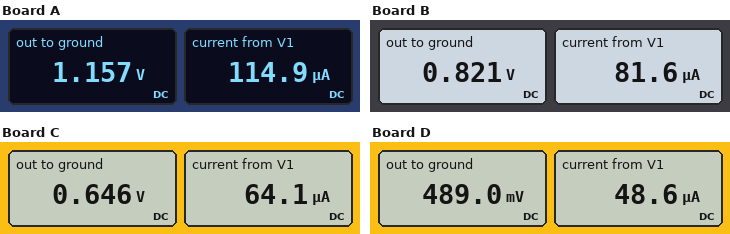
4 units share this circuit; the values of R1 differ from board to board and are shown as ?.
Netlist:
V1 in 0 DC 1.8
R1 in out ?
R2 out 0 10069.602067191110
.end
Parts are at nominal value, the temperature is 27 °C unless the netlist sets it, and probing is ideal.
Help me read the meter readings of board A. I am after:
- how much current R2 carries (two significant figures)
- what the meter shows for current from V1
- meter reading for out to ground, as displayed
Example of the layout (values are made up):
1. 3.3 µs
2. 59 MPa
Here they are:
1. 110 µA
2. 114.9 µA
3. 1.157 V
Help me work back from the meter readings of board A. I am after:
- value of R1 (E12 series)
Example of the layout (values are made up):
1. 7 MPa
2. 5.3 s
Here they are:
1. 5.6 kΩ
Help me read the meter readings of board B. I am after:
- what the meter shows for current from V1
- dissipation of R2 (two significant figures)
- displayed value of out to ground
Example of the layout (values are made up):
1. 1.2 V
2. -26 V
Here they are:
1. 81.6 µA
2. 67 µW
3. 0.821 V
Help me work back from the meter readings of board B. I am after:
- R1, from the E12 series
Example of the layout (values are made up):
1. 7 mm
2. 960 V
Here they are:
1. 12 kΩ
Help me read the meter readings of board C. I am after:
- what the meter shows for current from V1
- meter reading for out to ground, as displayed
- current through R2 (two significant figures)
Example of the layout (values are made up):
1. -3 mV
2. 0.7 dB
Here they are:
1. 64.1 µA
2. 0.646 V
3. 64 µA
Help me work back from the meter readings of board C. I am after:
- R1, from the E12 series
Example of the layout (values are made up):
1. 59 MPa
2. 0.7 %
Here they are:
1. 18 kΩ
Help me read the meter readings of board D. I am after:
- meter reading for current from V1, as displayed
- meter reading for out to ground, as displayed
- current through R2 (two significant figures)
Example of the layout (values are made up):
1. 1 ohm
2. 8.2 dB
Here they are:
1. 48.6 µA
2. 489.0 mV
3. 49 µA
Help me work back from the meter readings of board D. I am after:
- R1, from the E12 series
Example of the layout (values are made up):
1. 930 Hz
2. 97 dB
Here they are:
1. 27 kΩ
